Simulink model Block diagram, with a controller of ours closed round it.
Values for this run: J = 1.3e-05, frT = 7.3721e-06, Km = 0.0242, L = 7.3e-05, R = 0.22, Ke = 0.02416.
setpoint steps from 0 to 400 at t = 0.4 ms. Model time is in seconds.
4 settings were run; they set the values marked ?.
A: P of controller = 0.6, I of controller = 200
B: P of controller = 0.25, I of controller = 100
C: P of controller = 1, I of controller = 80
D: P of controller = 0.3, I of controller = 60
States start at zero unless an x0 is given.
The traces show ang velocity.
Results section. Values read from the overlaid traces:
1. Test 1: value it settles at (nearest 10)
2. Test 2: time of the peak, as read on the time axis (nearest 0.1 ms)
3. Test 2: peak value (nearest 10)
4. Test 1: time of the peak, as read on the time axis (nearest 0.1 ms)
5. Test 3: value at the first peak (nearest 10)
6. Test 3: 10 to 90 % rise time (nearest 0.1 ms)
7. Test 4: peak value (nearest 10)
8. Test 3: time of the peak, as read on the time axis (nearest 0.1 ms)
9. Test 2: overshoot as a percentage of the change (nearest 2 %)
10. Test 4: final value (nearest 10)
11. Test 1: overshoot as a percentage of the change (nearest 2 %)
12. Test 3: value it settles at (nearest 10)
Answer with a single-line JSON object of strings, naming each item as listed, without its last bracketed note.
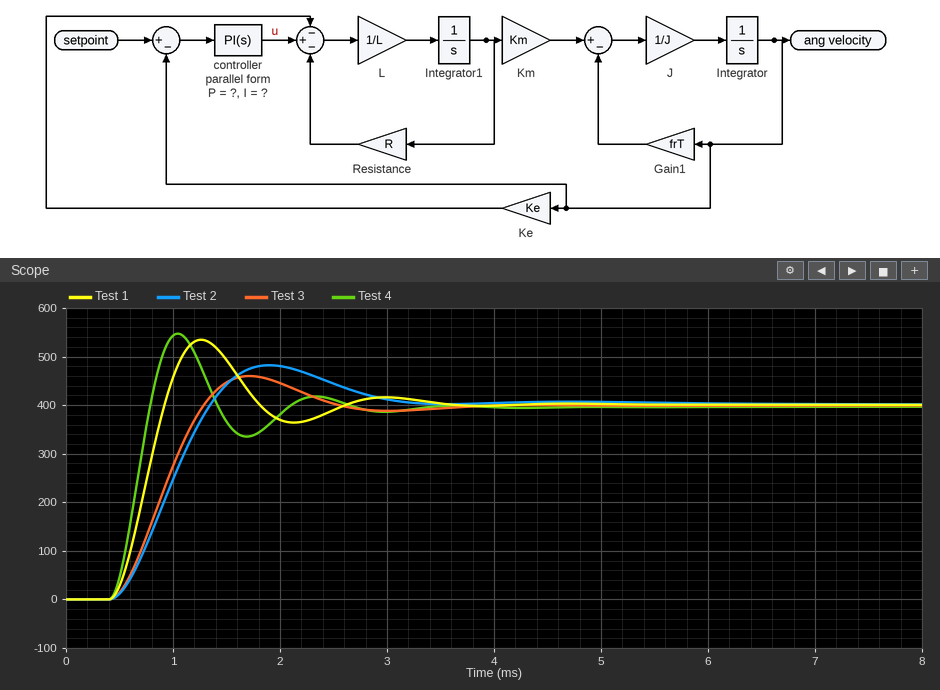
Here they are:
{"Test 1: value it settles at": "400", "Test 2: time of the peak, as read on the time axis": "1.9 ms", "Test 2: peak value": "480", "Test 1: time of the peak, as read on the time axis": "1.3 ms", "Test 3: value at the first peak": "460", "Test 3: 10 to 90 % rise time": "0.6 ms", "Test 4: peak value": "550", "Test 3: time of the peak, as read on the time axis": "1.7 ms", "Test 2: overshoot as a percentage of the change": "20 %", "Test 4: final value": "400", "Test 1: overshoot as a percentage of the change": "34 %", "Test 3: value it settles at": "400"}
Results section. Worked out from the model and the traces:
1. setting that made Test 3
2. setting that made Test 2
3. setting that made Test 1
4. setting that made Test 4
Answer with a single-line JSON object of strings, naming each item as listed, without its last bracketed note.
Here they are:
{"setting that made Test 3": "D", "setting that made Test 2": "B", "setting that made Test 1": "A", "setting that made Test 4": "C"}
